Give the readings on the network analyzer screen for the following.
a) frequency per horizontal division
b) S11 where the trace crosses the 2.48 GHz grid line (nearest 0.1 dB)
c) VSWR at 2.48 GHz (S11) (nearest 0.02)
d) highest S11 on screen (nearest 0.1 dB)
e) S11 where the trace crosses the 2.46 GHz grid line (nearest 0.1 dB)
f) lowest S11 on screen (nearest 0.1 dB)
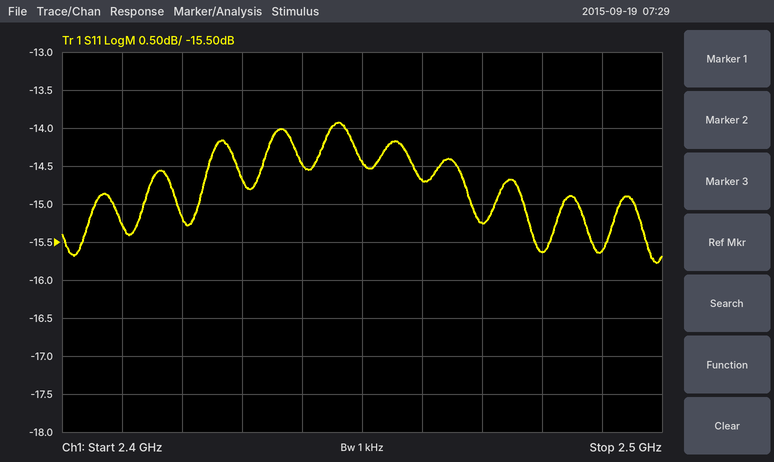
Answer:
10 MHz
-15.6 dB
1.40
-13.9 dB
-14.7 dB
-15.8 dB
